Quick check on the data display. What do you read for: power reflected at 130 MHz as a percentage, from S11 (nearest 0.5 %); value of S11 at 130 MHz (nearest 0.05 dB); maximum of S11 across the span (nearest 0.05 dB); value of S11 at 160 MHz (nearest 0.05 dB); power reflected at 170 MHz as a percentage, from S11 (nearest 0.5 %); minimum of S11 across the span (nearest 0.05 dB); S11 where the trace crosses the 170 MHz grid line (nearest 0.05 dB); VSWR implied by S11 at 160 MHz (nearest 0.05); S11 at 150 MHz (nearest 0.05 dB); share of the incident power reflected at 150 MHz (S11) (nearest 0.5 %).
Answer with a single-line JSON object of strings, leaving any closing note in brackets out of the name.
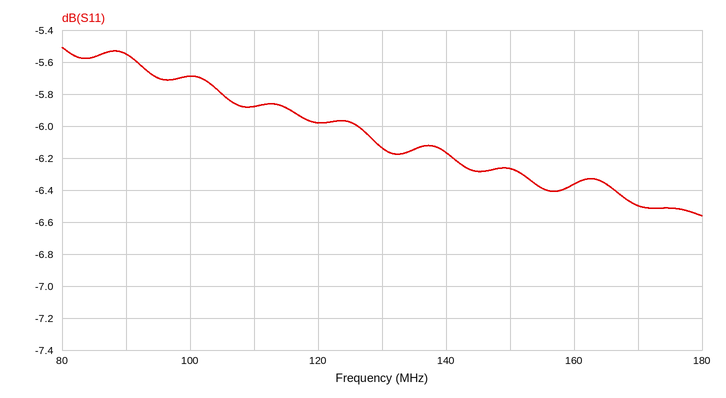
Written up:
{"power reflected at 130 MHz as a percentage, from S11": "24.5 %", "value of S11 at 130 MHz": "-6.15 dB", "maximum of S11 across the span": "-5.50 dB", "value of S11 at 160 MHz": "-6.35 dB", "power reflected at 170 MHz as a percentage, from S11": "22.5 %", "minimum of S11 across the span": "-6.55 dB", "S11 where the trace crosses the 170 MHz grid line": "-6.50 dB", "VSWR implied by S11 at 160 MHz": "2.85", "S11 at 150 MHz": "-6.25 dB", "share of the incident power reflected at 150 MHz (S11)": "23.5 %"}
